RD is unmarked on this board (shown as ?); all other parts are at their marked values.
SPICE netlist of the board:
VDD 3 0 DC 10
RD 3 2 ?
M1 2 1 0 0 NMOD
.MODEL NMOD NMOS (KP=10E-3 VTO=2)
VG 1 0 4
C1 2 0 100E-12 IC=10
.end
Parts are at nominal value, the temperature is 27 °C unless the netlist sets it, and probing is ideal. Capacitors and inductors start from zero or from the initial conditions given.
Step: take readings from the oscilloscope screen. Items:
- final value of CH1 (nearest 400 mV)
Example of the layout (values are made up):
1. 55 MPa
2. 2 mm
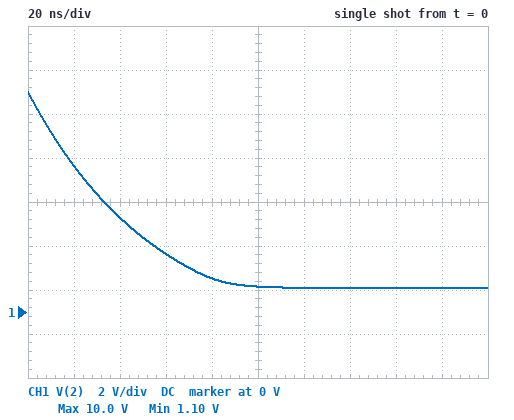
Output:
1. 1.2 V
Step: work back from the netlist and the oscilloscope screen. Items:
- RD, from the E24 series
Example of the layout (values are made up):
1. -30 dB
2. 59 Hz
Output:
1. 560 Ω
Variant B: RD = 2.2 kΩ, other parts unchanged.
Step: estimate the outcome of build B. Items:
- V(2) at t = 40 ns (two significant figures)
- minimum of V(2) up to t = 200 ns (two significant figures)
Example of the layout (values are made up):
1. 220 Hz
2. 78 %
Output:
1. 2.7 V
2. 240 mV
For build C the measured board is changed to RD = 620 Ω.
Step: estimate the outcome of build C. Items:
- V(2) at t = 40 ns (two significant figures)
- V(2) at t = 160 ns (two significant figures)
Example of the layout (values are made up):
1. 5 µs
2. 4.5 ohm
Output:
1. 4.1 V
2. 960 mV
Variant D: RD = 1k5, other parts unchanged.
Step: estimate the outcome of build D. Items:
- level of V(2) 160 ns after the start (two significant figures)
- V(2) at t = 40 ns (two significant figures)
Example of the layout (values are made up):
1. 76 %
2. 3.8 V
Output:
1. 350 mV
2. 3.0 V
